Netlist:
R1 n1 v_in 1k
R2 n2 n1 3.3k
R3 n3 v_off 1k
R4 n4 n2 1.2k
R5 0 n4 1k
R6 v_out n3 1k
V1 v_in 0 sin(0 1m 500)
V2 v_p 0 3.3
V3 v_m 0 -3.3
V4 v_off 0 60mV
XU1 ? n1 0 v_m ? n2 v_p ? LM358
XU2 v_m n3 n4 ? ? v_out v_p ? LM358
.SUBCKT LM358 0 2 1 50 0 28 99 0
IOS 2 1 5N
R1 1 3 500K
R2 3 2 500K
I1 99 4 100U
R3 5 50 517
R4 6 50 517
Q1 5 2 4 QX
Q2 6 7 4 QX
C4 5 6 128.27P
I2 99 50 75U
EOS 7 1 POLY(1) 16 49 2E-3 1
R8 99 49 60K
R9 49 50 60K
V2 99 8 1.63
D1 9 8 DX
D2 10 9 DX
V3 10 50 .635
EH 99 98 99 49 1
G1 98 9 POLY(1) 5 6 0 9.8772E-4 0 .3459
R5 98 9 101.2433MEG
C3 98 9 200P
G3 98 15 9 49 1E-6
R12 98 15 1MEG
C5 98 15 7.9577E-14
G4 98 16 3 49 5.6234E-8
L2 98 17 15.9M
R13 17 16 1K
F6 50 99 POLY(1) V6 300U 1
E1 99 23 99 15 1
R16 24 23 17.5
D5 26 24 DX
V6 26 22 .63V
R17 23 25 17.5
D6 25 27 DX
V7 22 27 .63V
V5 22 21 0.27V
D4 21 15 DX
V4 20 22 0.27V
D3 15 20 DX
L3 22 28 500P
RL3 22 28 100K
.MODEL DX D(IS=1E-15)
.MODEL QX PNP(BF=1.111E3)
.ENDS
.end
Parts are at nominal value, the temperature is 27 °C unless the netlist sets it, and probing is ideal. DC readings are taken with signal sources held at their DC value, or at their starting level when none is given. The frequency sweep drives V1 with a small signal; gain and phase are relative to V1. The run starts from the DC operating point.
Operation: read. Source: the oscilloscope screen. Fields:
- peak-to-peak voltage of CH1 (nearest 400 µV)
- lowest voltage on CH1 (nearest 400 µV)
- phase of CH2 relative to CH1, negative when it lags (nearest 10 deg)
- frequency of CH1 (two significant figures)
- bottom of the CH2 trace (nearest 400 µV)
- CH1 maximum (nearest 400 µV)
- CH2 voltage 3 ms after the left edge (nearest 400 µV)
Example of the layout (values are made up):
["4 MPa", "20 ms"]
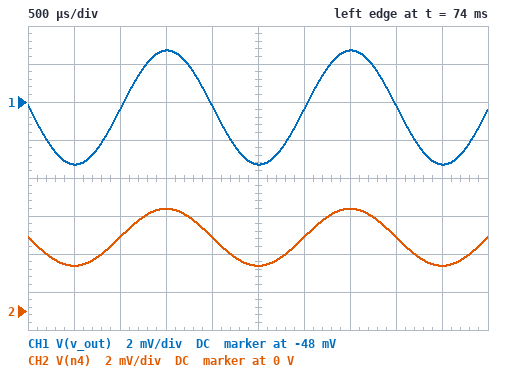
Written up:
["6.0 mV", "-51.2 mV", "0 deg", "500 Hz", "2.4 mV", "-45.2 mV", "4.0 mV"]
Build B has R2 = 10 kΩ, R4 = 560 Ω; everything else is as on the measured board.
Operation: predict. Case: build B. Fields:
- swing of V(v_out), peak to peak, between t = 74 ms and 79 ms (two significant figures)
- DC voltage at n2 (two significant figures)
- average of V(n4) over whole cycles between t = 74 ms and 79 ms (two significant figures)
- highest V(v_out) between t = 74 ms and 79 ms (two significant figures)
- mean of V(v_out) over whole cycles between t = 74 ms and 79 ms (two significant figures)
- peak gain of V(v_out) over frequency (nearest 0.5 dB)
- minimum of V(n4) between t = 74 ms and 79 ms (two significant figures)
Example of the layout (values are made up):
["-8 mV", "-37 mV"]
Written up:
["26 mV", "22 mV", "14 mV", "-15 mV", "-28 mV", "22.0 dB", "7.5 mV"]
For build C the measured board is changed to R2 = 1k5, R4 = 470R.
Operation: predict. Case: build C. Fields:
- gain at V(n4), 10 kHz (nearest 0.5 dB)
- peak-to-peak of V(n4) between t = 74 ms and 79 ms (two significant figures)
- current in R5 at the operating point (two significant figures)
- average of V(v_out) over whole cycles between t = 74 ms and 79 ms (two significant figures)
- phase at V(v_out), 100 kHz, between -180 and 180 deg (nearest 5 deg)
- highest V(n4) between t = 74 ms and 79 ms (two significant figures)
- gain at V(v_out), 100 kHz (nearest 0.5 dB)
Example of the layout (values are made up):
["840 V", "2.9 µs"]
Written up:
["0 dB", "2.0 mV", "3.4 µA", "-49 mV", "65 deg", "4.4 mV", "-10.0 dB"]
